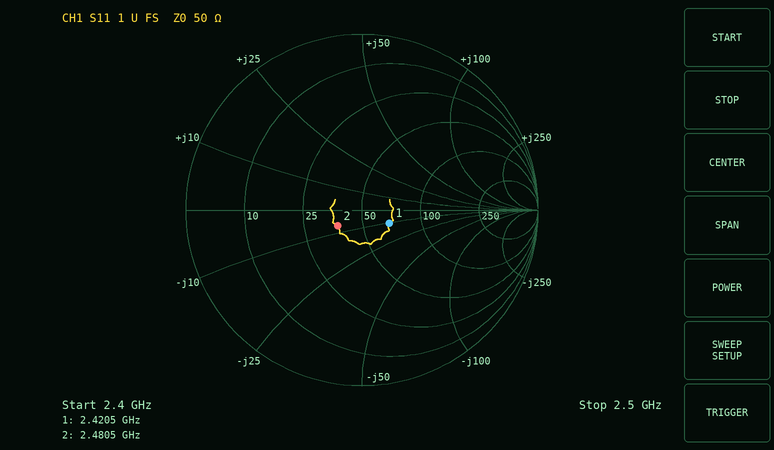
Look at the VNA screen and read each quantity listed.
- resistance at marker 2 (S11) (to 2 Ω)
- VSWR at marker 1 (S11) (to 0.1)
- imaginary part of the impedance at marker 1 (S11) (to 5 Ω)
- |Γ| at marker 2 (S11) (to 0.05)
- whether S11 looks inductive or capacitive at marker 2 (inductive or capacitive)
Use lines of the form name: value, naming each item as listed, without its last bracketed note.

resistance at marker 2 (S11): 38 Ω
VSWR at marker 1 (S11): 1.4
imaginary part of the impedance at marker 1 (S11): -10 Ω
|Γ| at marker 2 (S11): 0.15
whether S11 looks inductive or capacitive at marker 2: capacitive
